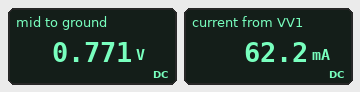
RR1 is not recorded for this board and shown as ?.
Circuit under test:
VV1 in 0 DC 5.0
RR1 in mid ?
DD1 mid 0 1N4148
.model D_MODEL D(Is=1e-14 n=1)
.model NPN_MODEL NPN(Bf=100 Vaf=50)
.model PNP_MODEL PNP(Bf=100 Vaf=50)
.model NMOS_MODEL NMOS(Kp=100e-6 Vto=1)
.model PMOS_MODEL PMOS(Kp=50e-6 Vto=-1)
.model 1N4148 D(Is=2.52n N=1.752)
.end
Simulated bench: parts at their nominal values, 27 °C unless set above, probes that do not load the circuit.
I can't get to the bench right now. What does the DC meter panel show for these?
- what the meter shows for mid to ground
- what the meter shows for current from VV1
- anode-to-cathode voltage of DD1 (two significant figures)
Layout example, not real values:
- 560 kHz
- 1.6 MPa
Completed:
- 0.771 V
- 62.2 mA
- 770 mV
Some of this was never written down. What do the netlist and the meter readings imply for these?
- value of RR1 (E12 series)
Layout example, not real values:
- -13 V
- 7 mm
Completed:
- 68 Ω
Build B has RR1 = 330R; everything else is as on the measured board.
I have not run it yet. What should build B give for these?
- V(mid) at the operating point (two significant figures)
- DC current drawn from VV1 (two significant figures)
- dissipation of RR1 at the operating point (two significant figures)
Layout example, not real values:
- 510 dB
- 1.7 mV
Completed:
- 700 mV
- 13 mA
- 56 mW
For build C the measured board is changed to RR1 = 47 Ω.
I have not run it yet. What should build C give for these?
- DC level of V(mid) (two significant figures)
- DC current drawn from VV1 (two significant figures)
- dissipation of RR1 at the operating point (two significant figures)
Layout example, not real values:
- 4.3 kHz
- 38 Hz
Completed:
- 790 mV
- 90 mA
- 380 mW
